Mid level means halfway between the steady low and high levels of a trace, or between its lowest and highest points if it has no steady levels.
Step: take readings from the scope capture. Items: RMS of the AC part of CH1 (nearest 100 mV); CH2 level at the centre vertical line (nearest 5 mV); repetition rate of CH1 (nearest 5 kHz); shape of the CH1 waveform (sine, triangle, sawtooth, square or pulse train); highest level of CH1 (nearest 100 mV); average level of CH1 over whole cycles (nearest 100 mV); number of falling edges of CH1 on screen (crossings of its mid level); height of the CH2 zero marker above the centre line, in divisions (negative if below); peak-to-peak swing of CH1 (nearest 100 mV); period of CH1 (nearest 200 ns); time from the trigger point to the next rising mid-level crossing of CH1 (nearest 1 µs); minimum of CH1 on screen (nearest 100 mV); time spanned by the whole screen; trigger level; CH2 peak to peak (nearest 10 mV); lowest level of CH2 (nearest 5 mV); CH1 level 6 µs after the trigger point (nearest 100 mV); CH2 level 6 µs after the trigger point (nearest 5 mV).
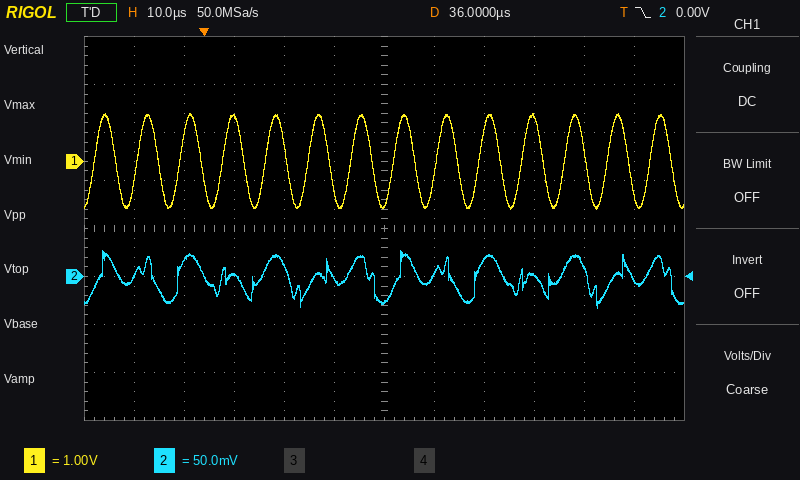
700 mV
-25 mV
115 kHz
sine
1.0 V
0.0 V
14
-1.0 div
2.0 V
8.6 µs
4 µs
-1.0 V
120 µs
0.00 V
60 mV
-35 mV
900 mV
0 mV
